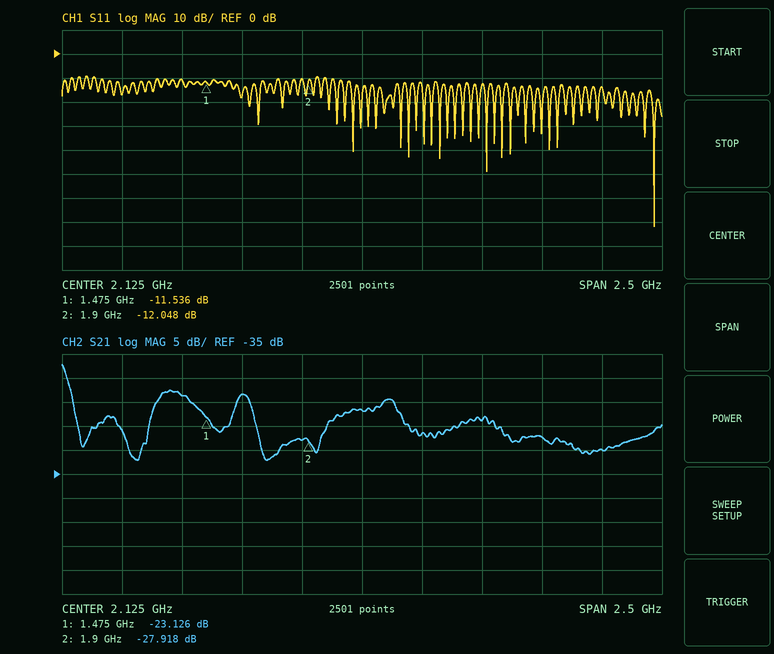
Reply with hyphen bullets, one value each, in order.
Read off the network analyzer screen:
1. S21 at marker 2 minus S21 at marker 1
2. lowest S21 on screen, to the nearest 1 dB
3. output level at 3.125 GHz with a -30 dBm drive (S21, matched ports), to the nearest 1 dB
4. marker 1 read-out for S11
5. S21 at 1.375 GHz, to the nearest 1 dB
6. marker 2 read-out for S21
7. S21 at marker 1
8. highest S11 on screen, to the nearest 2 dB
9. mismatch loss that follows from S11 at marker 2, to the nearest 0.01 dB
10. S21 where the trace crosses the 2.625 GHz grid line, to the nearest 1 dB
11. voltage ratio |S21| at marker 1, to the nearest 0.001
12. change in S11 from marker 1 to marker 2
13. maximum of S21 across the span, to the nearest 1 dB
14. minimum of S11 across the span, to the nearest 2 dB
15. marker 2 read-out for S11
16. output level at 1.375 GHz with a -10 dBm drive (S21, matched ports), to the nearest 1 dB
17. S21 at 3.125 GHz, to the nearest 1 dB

- -4.792 dB
- -32 dB
- -60 dBm
- -11.536 dB
- -19 dB
- -27.918 dB
- -23.126 dB
- -10 dB
- 0.28 dB
- -24 dB
- 0.070
- -0.512 dB
- -12 dB
- -72 dB
- -12.048 dB
- -29 dBm
- -30 dB
